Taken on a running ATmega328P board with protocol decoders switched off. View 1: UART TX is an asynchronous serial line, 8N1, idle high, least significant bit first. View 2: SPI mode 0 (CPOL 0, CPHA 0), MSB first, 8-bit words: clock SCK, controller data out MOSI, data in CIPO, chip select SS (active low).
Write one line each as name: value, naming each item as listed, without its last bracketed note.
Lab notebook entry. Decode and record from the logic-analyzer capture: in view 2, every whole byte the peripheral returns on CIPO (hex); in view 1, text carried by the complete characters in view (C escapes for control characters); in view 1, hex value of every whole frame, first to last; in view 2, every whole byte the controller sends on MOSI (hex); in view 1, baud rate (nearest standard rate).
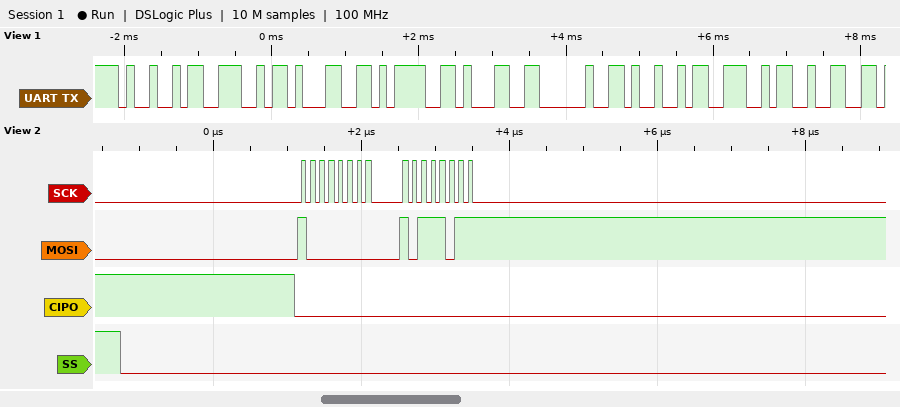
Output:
in view 2, every whole byte the peripheral returns on CIPO: 0x00 0x00
in view 1, text carried by the complete characters in view: "IN1=1 IN2"
in view 1, hex value of every whole frame, first to last: 49 4E 31 3D 31 20 49 4E 32
in view 2, every whole byte the controller sends on MOSI: 0x80 0xBB
in view 1, baud rate: 9600 baud
